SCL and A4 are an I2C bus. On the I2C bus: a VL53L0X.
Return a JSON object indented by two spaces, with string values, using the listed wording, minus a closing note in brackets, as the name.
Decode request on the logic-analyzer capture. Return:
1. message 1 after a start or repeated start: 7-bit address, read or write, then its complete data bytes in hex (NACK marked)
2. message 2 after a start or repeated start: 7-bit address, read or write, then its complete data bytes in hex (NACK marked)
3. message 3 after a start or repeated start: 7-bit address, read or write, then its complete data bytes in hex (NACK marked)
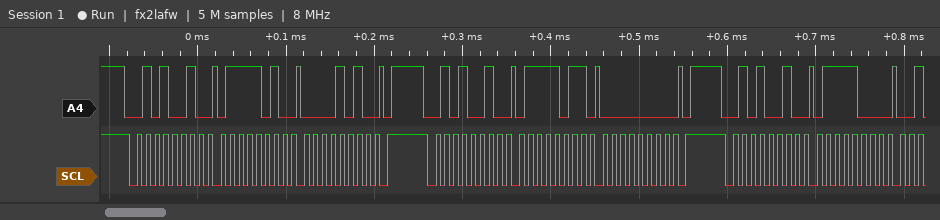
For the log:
{
  "message 1 after a start or repeated start: 7-bit address, read or write, then its complete data bytes in hex": "0x29 write: 7A 0A",
  "message 2 after a start or repeated start: 7-bit address, read or write, then its complete data bytes in hex": "0x29 write: 7B 00",
  "message 3 after a start or repeated start: 7-bit address, read or write, then its complete data bytes in hex": "0x29 write: 78"
}
